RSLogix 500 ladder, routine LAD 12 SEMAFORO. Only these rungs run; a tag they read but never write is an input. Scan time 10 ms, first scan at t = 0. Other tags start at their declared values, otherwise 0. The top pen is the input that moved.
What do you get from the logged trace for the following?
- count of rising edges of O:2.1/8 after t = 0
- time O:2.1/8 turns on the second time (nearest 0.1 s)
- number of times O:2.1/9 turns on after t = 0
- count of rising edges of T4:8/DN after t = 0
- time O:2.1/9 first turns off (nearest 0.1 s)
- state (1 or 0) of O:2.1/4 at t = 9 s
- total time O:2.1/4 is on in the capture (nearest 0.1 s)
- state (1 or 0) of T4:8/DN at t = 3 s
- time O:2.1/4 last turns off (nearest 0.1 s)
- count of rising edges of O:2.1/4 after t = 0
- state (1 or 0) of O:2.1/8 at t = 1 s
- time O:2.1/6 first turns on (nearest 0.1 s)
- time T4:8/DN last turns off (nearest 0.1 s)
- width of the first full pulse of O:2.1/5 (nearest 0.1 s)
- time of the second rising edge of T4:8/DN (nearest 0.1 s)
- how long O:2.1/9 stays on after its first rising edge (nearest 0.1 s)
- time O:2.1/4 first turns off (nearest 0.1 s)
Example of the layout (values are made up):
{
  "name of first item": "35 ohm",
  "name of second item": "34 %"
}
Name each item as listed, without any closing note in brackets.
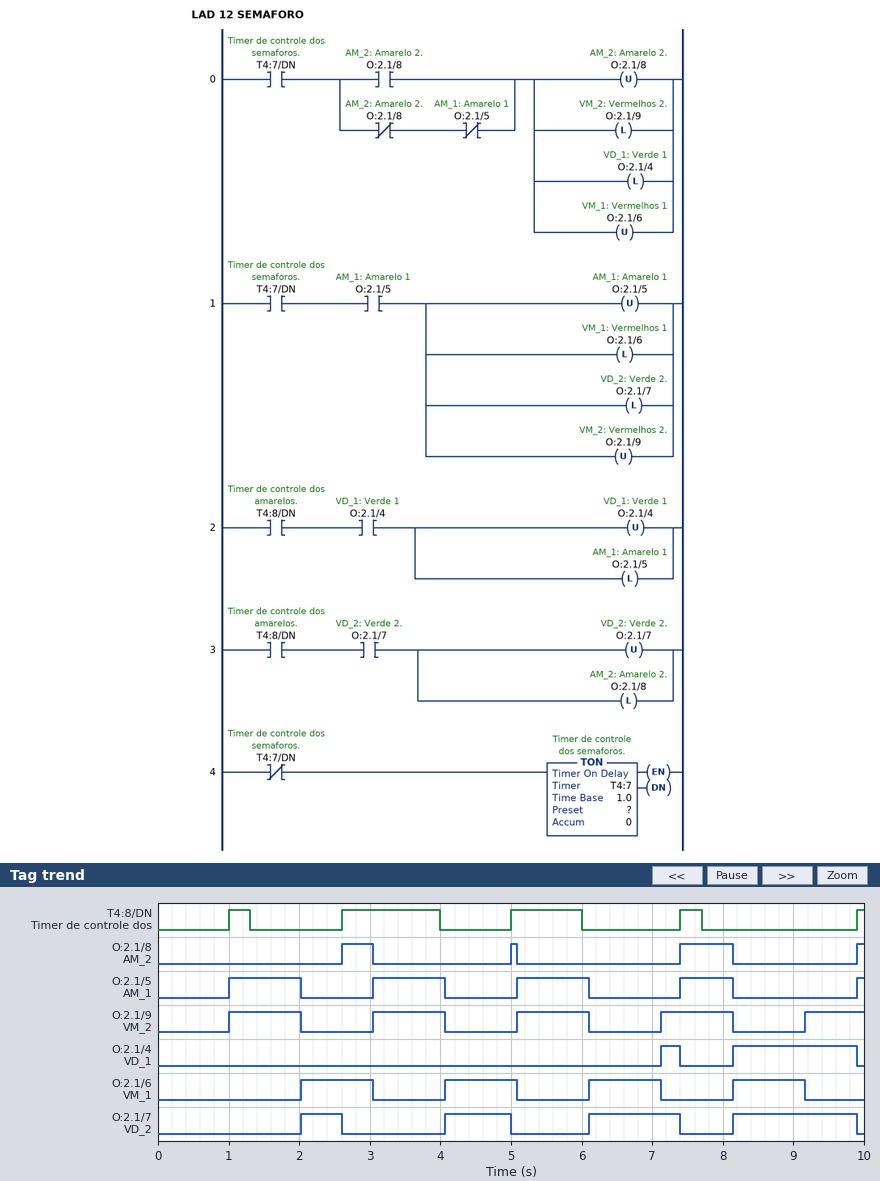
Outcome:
{
  "count of rising edges of O:2.1/8 after t = 0": "4",
  "time O:2.1/8 turns on the second time": "5.0 s",
  "number of times O:2.1/9 turns on after t = 0": "5",
  "count of rising edges of T4:8/DN after t = 0": "5",
  "time O:2.1/9 first turns off": "2.0 s",
  "state (1 or 0) of O:2.1/4 at t = 9 s": "1",
  "total time O:2.1/4 is on in the capture": "2.0 s",
  "state (1 or 0) of T4:8/DN at t = 3 s": "1",
  "time O:2.1/4 last turns off": "9.9 s",
  "count of rising edges of O:2.1/4 after t = 0": "2",
  "state (1 or 0) of O:2.1/8 at t = 1 s": "0",
  "time O:2.1/6 first turns on": "2.0 s",
  "time T4:8/DN last turns off": "7.7 s",
  "width of the first full pulse of O:2.1/5": "1.0 s",
  "time of the second rising edge of T4:8/DN": "2.6 s",
  "how long O:2.1/9 stays on after its first rising edge": "1.0 s",
  "time O:2.1/4 first turns off": "7.4 s"
}
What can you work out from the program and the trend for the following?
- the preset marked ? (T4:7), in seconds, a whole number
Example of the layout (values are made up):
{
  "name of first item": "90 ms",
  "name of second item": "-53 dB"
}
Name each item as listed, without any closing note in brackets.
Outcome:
{
  "the preset marked ? (T4:7), in seconds, a whole number": "1 s"
}
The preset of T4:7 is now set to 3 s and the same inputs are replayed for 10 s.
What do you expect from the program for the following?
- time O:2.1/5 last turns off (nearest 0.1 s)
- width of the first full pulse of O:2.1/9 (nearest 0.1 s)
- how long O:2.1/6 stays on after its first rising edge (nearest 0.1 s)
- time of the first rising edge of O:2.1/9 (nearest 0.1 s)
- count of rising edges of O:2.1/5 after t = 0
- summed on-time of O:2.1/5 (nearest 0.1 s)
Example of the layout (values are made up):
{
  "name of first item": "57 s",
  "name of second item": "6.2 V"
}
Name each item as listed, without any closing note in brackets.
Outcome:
{
  "time O:2.1/5 last turns off": "6.0 s",
  "width of the first full pulse of O:2.1/9": "3.0 s",
  "how long O:2.1/6 stays on after its first rising edge": "3.0 s",
  "time of the first rising edge of O:2.1/9": "3.0 s",
  "count of rising edges of O:2.1/5 after t = 0": "2",
  "summed on-time of O:2.1/5": "3.1 s"
}
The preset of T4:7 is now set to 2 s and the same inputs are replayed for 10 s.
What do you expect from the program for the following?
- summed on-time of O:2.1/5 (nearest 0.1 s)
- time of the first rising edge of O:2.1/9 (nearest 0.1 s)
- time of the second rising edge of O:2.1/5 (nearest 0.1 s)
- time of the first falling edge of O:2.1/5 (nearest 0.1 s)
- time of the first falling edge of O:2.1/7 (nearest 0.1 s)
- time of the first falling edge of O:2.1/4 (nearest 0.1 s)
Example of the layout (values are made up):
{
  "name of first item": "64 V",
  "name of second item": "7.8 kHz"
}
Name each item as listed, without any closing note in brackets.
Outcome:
{
  "summed on-time of O:2.1/5": "2.1 s",
  "time of the first rising edge of O:2.1/9": "2.0 s",
  "time of the second rising edge of O:2.1/5": "7.4 s",
  "time of the first falling edge of O:2.1/5": "4.0 s",
  "time of the first falling edge of O:2.1/7": "5.0 s",
  "time of the first falling edge of O:2.1/4": "2.6 s"
}
